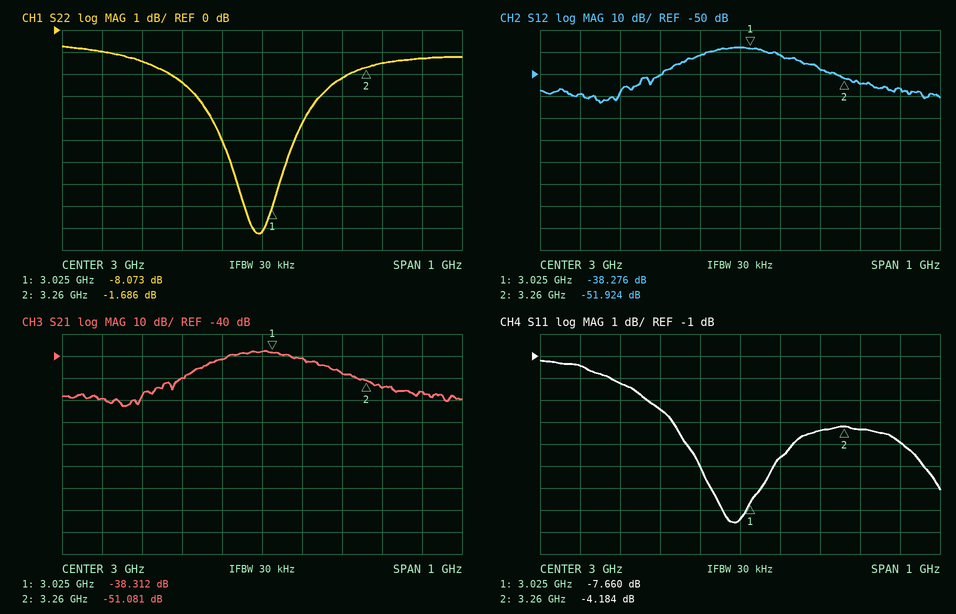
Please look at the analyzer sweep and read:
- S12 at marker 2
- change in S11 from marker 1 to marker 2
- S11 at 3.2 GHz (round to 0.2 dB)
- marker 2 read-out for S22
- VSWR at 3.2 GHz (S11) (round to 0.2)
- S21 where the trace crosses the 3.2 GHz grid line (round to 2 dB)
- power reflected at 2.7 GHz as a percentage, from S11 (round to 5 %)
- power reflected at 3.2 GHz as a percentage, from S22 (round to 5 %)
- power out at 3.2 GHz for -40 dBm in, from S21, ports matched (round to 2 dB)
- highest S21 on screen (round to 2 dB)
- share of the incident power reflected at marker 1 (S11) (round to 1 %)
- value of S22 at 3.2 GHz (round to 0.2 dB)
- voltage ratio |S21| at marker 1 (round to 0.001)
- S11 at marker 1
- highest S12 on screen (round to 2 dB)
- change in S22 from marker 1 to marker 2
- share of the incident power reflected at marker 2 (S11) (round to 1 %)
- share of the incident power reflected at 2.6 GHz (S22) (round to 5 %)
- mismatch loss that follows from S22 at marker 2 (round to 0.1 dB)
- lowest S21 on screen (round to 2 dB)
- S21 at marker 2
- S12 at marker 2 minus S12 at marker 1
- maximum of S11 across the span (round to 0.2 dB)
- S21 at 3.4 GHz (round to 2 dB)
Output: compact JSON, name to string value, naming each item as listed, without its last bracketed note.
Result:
{"S12 at marker 2": "-51.924 dB", "change in S11 from marker 1 to marker 2": "3.476 dB", "S11 at 3.2 GHz": "-4.4 dB", "marker 2 read-out for S22": "-1.686 dB", "VSWR at 3.2 GHz (S11)": "4.0", "S21 where the trace crosses the 3.2 GHz grid line": "-48 dB", "power reflected at 2.7 GHz as a percentage, from S11": "60 %", "power reflected at 3.2 GHz as a percentage, from S22": "60 %", "power out at 3.2 GHz for -40 dBm in, from S21, ports matched": "-88 dBm", "highest S21 on screen": "-38 dB", "share of the incident power reflected at marker 1 (S11)": "17 %", "value of S22 at 3.2 GHz": "-2.2 dB", "voltage ratio |S21| at marker 1": "0.012", "S11 at marker 1": "-7.660 dB", "highest S12 on screen": "-38 dB", "change in S22 from marker 1 to marker 2": "6.387 dB", "share of the incident power reflected at marker 2 (S11)": "38 %", "share of the incident power reflected at 2.6 GHz (S22)": "80 %", "mismatch loss that follows from S22 at marker 2": "4.9 dB", "lowest S21 on screen": "-62 dB", "S21 at marker 2": "-51.081 dB", "S12 at marker 2 minus S12 at marker 1": "-13.648 dB", "maximum of S11 across the span": "-1.2 dB", "S21 at 3.4 GHz": "-56 dB"}
